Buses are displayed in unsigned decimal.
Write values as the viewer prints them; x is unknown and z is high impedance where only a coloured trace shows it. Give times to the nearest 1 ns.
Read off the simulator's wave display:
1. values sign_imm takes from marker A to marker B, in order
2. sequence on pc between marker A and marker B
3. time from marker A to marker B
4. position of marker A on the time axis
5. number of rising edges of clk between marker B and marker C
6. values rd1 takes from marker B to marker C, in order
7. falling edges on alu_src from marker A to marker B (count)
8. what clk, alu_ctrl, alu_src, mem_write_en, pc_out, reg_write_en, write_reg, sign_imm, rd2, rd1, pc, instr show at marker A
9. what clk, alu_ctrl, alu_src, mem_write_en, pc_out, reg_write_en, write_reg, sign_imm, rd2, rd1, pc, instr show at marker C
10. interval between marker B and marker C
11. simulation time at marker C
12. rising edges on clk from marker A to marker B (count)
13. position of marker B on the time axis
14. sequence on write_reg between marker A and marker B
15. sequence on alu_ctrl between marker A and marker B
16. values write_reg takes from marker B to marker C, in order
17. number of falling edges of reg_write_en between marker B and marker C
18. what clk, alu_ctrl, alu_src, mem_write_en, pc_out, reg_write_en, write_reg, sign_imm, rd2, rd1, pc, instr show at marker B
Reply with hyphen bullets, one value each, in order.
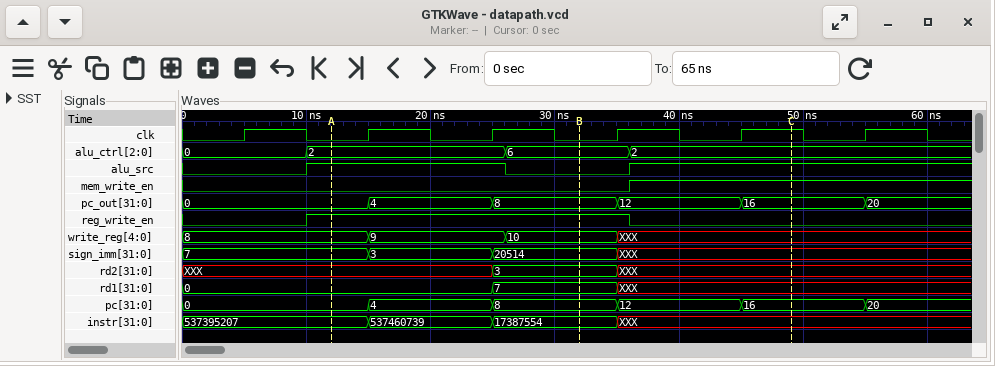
- 7, 3, 20514
- 0, 4, 8
- 20 ns
- 12 ns
- 2
- 7, XXX
- 1
- clk=0, alu_ctrl=2, alu_src=1, mem_write_en=0, pc_out=0, reg_write_en=1, write_reg=8, sign_imm=7, rd2=XXX, rd1=0, pc=0, instr=537395207
- clk=1, alu_ctrl=2, alu_src=1, mem_write_en=1, pc_out=16, reg_write_en=0, write_reg=XXX, sign_imm=XXX, rd2=XXX, rd1=XXX, pc=16, instr=XXX
- 17 ns
- 49 ns
- 2
- 32 ns
- 8, 9, 10
- 2, 6
- 10, XXX
- 1
- clk=0, alu_ctrl=6, alu_src=0, mem_write_en=0, pc_out=8, reg_write_en=1, write_reg=10, sign_imm=20514, rd2=3, rd1=7, pc=8, instr=17387554
